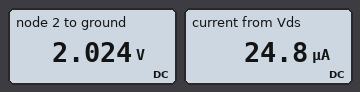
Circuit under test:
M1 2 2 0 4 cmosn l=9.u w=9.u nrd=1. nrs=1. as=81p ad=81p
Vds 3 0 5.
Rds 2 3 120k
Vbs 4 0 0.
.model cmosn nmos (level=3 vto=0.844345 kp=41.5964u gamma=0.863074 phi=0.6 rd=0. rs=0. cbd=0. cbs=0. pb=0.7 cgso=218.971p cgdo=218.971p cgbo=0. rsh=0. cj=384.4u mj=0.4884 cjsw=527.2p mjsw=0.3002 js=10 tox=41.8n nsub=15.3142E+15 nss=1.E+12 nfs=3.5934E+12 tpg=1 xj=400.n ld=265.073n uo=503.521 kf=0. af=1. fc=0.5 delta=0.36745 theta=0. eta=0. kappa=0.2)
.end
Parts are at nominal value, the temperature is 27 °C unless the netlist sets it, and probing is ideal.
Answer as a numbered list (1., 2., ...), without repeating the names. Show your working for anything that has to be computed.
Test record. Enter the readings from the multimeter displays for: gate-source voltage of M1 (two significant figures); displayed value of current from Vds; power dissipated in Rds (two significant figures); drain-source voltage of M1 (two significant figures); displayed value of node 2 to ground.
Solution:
1. 2.024 V = 2.0 V
2. 24.8 µA
3. (5 V - 2.024 V)^2 / 120 kΩ = 74 µW
4. 2.024 V = 2.0 V
5. 2.024 V
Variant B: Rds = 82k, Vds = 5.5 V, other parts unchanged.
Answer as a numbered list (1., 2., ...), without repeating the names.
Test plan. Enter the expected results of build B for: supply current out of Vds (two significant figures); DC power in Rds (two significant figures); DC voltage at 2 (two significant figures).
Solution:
1. 39 µA
2. 120 µW
3. 2.3 V
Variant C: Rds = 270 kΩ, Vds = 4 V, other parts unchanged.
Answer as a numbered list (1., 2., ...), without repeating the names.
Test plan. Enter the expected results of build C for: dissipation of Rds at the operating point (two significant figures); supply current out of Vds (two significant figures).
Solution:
1. 22 µW
2. 9.1 µA
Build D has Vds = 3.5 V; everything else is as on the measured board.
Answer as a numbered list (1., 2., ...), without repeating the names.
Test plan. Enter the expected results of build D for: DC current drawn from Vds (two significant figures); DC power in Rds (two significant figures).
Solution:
1. 15 µA
2. 26 µW
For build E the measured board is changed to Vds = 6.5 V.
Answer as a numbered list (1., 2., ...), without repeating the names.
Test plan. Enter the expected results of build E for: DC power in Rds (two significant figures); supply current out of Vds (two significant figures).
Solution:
1. 150 µW
2. 35 µA
